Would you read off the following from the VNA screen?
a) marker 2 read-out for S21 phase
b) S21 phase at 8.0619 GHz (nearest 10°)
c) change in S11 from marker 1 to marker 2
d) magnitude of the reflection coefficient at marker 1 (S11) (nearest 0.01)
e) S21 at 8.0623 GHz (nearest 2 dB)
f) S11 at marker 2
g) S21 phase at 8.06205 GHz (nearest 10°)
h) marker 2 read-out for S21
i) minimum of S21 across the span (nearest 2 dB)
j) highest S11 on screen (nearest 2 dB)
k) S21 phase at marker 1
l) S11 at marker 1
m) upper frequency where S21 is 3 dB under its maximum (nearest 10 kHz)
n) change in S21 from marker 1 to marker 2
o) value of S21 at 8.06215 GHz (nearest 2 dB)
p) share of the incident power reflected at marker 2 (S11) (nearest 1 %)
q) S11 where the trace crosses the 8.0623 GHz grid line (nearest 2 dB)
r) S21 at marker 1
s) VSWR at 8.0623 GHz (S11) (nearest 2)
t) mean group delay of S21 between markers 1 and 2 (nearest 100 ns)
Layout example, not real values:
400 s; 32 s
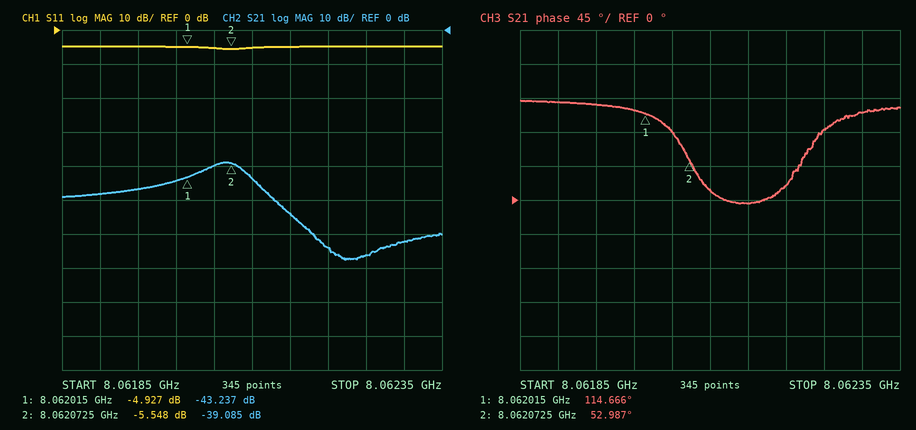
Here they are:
52.987°; 130°; -0.621 dB; 0.57; -62 dB; -5.548 dB; 90°; -39.085 dB; -68 dB; -4 dB; 114.666°; -4.927 dB; 8.06209 GHz; 4.152 dB; -54 dB; 28 %; -4 dB; -43.237 dB; 4; 3.0 µs
